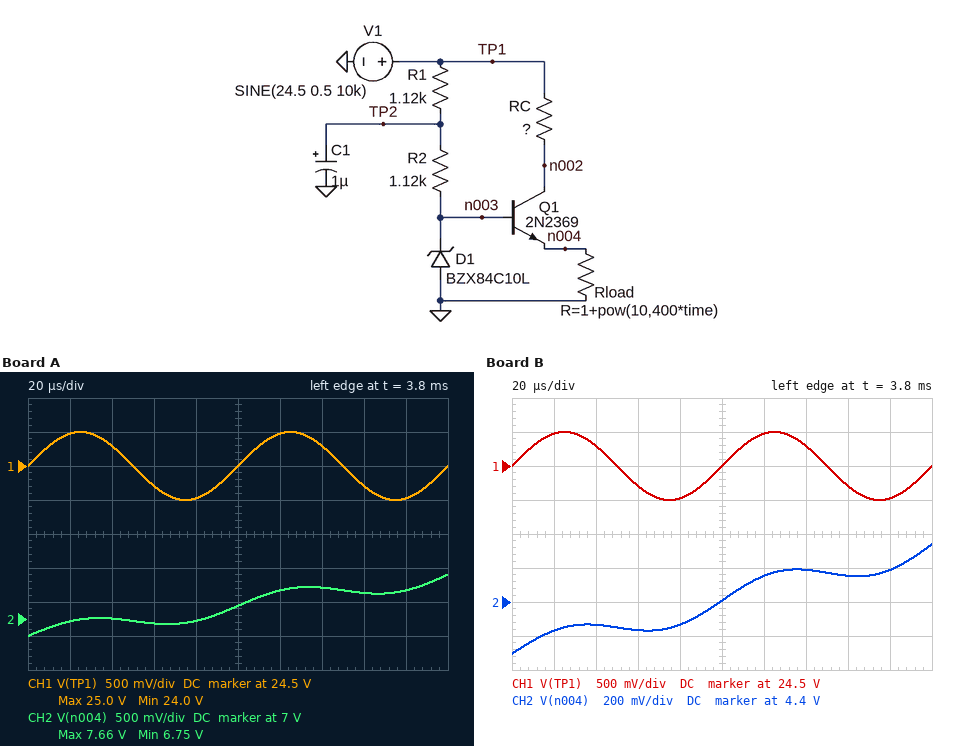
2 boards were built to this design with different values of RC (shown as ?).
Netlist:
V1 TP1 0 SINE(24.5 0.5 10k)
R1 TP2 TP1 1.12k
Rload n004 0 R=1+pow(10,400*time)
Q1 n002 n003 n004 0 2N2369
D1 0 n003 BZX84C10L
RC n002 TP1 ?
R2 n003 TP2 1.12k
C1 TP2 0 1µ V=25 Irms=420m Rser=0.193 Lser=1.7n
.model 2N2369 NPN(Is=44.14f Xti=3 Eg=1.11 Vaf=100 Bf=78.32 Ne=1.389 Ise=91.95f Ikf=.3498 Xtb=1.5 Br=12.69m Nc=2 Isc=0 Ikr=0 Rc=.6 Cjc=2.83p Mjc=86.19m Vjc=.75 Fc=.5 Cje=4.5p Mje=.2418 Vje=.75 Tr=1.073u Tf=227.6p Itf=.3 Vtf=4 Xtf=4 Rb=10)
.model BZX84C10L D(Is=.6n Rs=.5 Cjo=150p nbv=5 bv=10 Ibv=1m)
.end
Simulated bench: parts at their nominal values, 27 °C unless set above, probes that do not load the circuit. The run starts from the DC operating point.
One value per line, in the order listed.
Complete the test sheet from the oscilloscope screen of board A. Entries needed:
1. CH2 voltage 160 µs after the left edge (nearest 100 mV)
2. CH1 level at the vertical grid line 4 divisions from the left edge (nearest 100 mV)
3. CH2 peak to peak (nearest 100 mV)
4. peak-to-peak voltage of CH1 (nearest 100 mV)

7.4 V
24.0 V
900 mV
1.0 V
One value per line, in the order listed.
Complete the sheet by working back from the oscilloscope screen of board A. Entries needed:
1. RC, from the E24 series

91 Ω
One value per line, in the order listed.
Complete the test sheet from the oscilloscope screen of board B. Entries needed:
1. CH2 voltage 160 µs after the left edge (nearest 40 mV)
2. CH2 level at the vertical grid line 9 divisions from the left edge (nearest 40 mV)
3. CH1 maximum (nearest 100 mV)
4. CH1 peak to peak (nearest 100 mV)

4.56 V
4.60 V
25.0 V
1.0 V
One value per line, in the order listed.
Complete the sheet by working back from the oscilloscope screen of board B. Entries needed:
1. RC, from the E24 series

180 Ω
